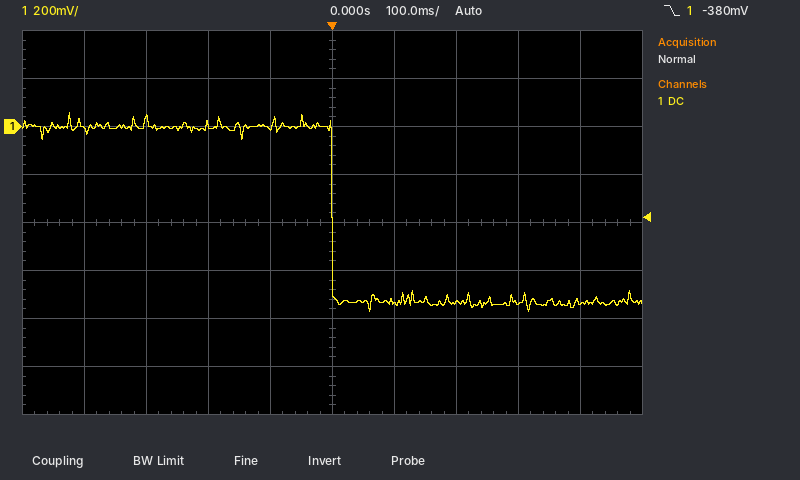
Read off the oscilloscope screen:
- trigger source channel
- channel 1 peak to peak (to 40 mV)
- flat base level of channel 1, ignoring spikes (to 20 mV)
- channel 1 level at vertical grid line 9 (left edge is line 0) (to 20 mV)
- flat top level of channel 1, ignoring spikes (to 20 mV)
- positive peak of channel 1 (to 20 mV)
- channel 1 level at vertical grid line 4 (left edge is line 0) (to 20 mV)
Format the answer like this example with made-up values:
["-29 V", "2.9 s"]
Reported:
["channel 1", "840 mV", "-740 mV", "-720 mV", "0 mV", "60 mV", "0 mV"]
